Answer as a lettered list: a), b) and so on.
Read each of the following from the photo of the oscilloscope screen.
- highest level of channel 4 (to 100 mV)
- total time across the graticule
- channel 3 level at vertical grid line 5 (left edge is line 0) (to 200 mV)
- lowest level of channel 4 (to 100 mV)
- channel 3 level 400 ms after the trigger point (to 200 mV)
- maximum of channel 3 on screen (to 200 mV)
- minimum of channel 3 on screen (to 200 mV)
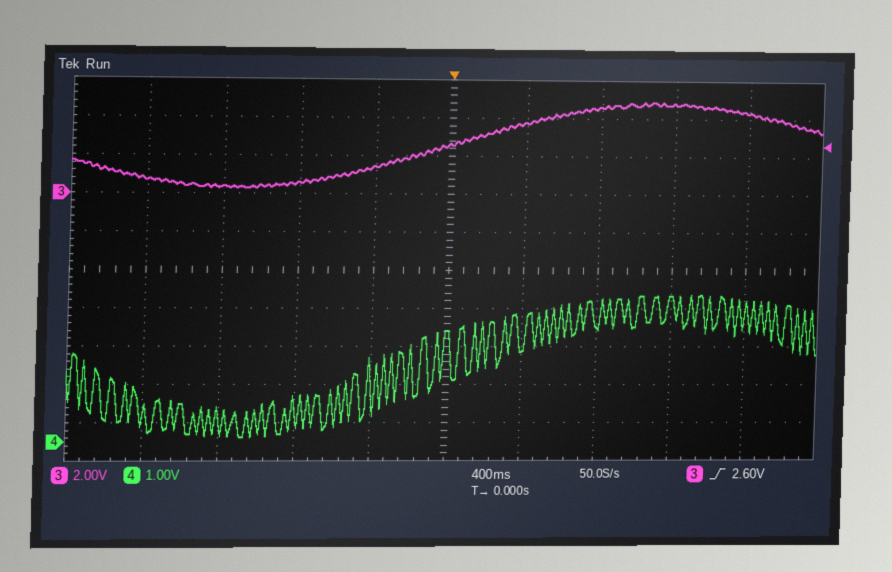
a) 3.9 V
b) 4 s
c) 2.6 V
d) 100 mV
e) 3.8 V
f) 4.8 V
g) 400 mV
